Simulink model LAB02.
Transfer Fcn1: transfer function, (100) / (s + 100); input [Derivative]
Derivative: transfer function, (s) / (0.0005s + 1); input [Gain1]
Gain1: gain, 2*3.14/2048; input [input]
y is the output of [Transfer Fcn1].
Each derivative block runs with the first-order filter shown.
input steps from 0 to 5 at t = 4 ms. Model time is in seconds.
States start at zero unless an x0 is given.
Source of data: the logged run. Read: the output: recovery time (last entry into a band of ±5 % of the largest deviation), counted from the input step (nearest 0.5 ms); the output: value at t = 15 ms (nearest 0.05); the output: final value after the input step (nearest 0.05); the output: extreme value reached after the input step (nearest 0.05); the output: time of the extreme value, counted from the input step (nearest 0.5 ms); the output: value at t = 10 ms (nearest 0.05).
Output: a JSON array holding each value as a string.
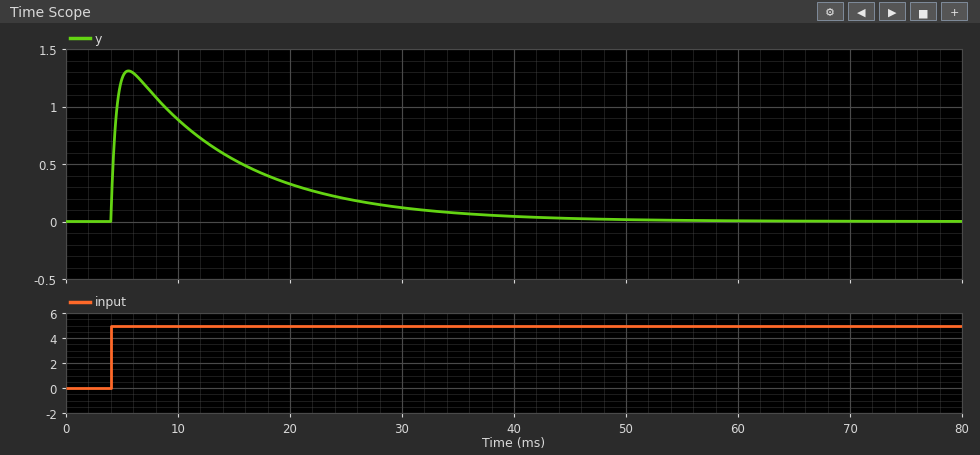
["32.0 ms", "0.55", "0.00", "1.30", "1.5 ms", "0.90"]
